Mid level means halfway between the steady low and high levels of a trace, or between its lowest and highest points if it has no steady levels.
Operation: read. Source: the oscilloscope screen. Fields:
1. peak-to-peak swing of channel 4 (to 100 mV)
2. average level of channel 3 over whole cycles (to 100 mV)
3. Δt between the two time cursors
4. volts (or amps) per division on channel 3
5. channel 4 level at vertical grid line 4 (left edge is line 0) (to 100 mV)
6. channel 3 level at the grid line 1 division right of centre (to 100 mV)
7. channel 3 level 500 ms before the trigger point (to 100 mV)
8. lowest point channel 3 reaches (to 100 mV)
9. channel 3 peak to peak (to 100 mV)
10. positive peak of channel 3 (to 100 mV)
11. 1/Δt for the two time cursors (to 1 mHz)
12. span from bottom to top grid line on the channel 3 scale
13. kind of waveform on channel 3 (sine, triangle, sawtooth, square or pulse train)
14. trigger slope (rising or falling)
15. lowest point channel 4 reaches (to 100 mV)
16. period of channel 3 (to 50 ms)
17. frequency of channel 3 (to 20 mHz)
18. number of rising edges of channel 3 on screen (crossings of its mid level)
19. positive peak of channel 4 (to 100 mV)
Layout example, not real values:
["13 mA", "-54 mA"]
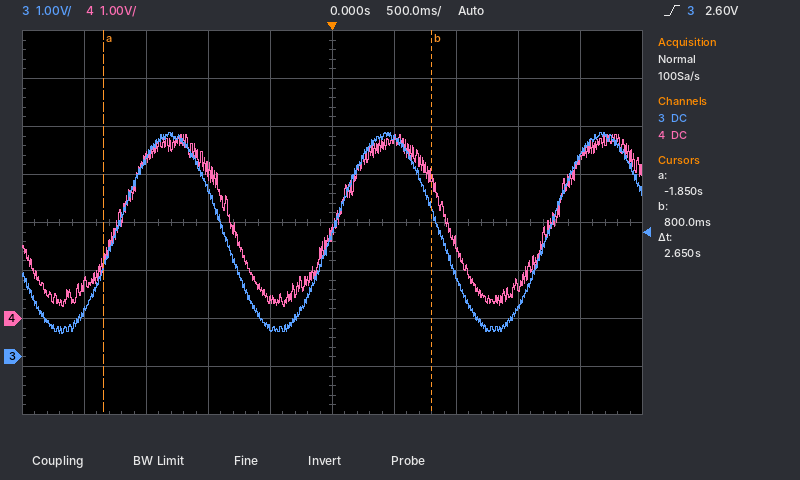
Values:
["3.6 V", "2.6 V", "2.65 s", "1 V", "400 mV", "4.6 V", "600 mV", "500 mV", "4.2 V", "4.7 V", "377 mHz", "8 V", "sine", "rising", "200 mV", "1.75 s", "580 mHz", "3", "3.8 V"]
